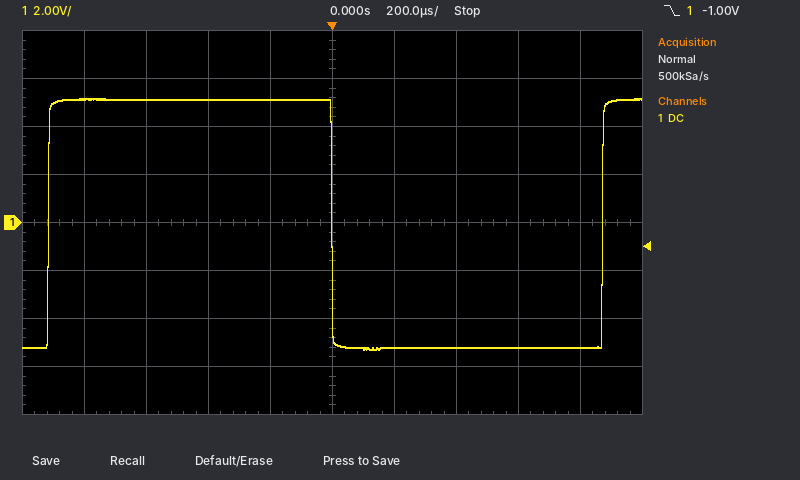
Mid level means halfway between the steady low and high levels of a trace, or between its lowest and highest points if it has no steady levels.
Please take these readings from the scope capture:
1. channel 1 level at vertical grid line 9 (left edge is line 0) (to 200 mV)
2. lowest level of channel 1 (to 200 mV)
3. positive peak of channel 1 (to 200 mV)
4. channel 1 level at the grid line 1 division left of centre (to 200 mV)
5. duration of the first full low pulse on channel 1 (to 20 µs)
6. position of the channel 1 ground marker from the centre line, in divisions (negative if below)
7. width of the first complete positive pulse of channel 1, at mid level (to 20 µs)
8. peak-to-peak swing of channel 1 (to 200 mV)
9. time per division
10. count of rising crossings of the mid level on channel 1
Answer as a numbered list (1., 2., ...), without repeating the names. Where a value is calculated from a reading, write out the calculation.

1. -5.2 V
2. -5.2 V
3. 5.2 V
4. 5.2 V
5. 880 µs
6. 0.0 div
7. 920 µs
8. 5.2 V − (-5.2 V) = 10.4 V
9. 200 µs
10. 2
